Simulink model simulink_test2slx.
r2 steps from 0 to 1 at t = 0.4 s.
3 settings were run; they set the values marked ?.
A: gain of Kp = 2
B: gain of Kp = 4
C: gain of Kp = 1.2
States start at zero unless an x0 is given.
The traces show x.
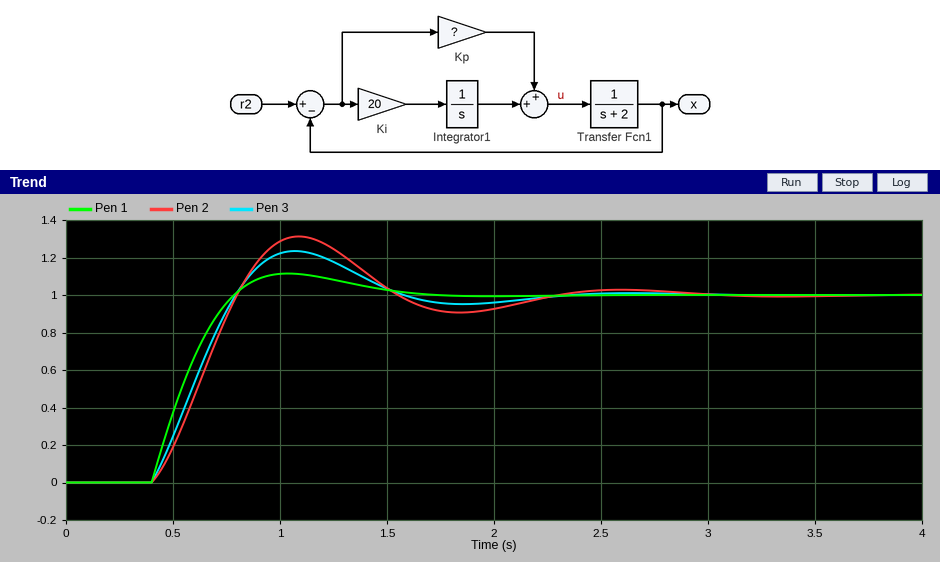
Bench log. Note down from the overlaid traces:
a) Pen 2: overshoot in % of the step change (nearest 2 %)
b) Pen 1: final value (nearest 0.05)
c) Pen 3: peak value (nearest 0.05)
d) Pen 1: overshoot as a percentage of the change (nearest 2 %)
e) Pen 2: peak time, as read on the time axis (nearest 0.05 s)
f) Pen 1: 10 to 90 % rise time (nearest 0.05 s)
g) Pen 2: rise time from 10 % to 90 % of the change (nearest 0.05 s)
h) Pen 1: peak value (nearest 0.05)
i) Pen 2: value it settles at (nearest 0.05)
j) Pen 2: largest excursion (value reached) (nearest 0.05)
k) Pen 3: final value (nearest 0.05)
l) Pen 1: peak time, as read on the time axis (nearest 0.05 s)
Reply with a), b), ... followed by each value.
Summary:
a) 32 %
b) 1.00
c) 1.25
d) 12 %
e) 1.10 s
f) 0.30 s
g) 0.30 s
h) 1.10
i) 1.00
j) 1.30
k) 1.00
l) 1.05 s
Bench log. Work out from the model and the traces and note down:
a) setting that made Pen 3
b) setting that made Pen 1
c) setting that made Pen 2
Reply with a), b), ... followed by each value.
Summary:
a) A
b) B
c) C
